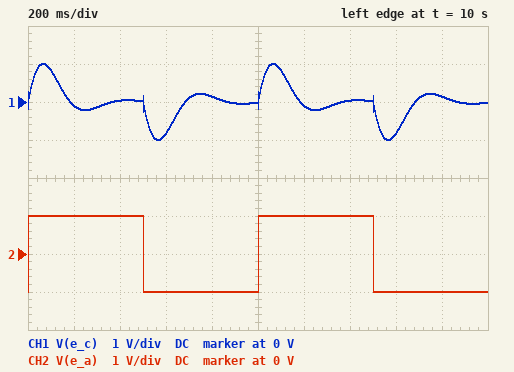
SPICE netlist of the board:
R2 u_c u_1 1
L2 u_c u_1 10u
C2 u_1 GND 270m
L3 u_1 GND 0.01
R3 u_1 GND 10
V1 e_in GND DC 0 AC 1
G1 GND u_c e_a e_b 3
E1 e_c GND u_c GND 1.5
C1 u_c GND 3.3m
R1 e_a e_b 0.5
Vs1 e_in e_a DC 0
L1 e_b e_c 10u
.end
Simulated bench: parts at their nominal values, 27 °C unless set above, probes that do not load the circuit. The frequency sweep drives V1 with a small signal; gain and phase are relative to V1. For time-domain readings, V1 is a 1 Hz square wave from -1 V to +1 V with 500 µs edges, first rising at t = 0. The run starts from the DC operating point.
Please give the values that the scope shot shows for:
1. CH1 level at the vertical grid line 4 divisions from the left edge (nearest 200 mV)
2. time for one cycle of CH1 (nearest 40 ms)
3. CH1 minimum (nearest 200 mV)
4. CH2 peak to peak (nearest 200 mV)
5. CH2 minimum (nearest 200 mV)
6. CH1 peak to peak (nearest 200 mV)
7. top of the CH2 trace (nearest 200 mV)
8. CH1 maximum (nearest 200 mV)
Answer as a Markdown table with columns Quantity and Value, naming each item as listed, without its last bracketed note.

| Quantity | Value |
|---|---|
| CH1 level at the vertical grid line 4 divisions from the left edge | 200 mV |
| time for one cycle of CH1 | 1.00 s |
| CH1 minimum | -1.0 V |
| CH2 peak to peak | 2.0 V |
| CH2 minimum | -1.0 V |
| CH1 peak to peak | 2.0 V |
| top of the CH2 trace | 1.0 V |
| CH1 maximum | 1.0 V |
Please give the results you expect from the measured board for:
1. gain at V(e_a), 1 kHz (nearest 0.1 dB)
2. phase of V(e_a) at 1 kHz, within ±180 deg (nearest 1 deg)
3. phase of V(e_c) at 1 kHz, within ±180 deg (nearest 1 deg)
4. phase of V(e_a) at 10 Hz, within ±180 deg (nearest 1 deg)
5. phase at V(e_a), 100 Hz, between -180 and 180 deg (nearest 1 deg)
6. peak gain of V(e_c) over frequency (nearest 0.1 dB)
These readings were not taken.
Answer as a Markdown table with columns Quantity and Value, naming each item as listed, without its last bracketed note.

| Quantity | Value |
|---|---|
| gain at V(e_a), 1 kHz | 0 dB |
| phase of V(e_a) at 1 kHz, within ±180 deg | 0 deg |
| phase of V(e_c) at 1 kHz, within ±180 deg | -44 deg |
| phase of V(e_a) at 10 Hz, within ±180 deg | 0 deg |
| phase at V(e_a), 100 Hz, between -180 and 180 deg | 0 deg |
| peak gain of V(e_c) over frequency | -0.2 dB |
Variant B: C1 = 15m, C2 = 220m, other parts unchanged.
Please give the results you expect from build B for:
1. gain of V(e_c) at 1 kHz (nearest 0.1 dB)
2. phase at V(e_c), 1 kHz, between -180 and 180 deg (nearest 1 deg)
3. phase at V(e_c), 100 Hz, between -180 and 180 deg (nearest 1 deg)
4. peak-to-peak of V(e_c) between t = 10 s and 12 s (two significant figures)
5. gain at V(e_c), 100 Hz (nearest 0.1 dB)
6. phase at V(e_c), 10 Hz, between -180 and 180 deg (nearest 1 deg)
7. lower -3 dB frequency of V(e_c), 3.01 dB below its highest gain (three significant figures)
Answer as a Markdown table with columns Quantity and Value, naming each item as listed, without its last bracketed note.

| Quantity | Value |
|---|---|
| gain of V(e_c) at 1 kHz | -24.8 dB |
| phase at V(e_c), 1 kHz, between -180 and 180 deg | -93 deg |
| phase at V(e_c), 100 Hz, between -180 and 180 deg | -88 deg |
| peak-to-peak of V(e_c) between t = 10 s and 12 s | 2.1 V |
| gain at V(e_c), 100 Hz | -47.4 dB |
| phase at V(e_c), 10 Hz, between -180 and 180 deg | -71 deg |
| lower -3 dB frequency of V(e_c), 3.01 dB below its highest gain | 2.08 Hz |
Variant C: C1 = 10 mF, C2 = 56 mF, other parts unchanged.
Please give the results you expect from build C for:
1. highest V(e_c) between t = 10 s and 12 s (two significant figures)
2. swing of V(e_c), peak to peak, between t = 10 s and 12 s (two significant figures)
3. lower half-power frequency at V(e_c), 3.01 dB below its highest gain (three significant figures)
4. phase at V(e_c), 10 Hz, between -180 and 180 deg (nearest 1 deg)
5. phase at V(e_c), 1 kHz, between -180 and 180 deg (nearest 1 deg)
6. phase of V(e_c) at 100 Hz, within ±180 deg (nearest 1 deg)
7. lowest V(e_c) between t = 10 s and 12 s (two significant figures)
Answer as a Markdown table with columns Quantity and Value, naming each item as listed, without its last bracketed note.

| Quantity | Value |
|---|---|
| highest V(e_c) between t = 10 s and 12 s | 1.4 V |
| swing of V(e_c), peak to peak, between t = 10 s and 12 s | 2.8 V |
| lower half-power frequency at V(e_c), 3.01 dB below its highest gain | 2.77 Hz |
| phase at V(e_c), 10 Hz, between -180 and 180 deg | -29 deg |
| phase at V(e_c), 1 kHz, between -180 and 180 deg | -90 deg |
| phase of V(e_c) at 100 Hz, within ±180 deg | -85 deg |
| lowest V(e_c) between t = 10 s and 12 s | -1.4 V |
